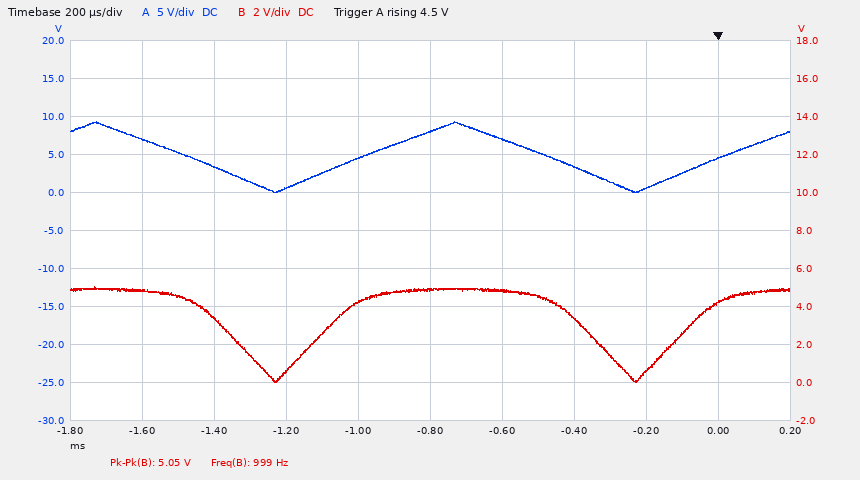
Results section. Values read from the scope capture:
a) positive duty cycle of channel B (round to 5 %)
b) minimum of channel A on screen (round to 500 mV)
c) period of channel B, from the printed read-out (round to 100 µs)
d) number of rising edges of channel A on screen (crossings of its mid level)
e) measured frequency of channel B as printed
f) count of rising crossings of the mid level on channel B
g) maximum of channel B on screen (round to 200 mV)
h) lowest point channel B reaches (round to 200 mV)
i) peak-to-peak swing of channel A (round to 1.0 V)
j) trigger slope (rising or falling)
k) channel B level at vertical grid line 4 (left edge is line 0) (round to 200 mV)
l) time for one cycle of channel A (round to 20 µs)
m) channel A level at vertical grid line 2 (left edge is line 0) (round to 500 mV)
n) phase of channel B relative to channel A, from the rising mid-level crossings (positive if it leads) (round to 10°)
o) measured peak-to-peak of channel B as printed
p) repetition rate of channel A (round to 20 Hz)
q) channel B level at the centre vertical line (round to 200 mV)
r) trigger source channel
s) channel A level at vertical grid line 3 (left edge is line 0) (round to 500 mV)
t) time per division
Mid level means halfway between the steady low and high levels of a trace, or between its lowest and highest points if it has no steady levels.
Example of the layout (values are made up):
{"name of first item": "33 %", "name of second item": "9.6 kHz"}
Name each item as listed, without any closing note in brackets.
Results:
{"positive duty cycle of channel B": "75 %", "minimum of channel A on screen": "0.0 V", "period of channel B, from the printed read-out": "1.0 ms", "number of rising edges of channel A on screen": "2", "measured frequency of channel B as printed": "999 Hz", "count of rising crossings of the mid level on channel B": "2", "maximum of channel B on screen": "5.0 V", "lowest point channel B reaches": "0.0 V", "peak-to-peak swing of channel A": "9.0 V", "trigger slope": "rising", "channel B level at vertical grid line 4 (left edge is line 0)": "4.2 V", "time for one cycle of channel A": "1.00 ms", "channel A level at vertical grid line 2 (left edge is line 0)": "3.5 V", "phase of channel B relative to channel A, from the rising mid-level crossings (positive if it leads)": "+40°", "measured peak-to-peak of channel B as printed": "5.05 V", "repetition rate of channel A": "1.00 kHz", "channel B level at the centre vertical line": "4.8 V", "trigger source channel": "channel A", "channel A level at vertical grid line 3 (left edge is line 0)": "500 mV", "time per division": "200 µs"}
